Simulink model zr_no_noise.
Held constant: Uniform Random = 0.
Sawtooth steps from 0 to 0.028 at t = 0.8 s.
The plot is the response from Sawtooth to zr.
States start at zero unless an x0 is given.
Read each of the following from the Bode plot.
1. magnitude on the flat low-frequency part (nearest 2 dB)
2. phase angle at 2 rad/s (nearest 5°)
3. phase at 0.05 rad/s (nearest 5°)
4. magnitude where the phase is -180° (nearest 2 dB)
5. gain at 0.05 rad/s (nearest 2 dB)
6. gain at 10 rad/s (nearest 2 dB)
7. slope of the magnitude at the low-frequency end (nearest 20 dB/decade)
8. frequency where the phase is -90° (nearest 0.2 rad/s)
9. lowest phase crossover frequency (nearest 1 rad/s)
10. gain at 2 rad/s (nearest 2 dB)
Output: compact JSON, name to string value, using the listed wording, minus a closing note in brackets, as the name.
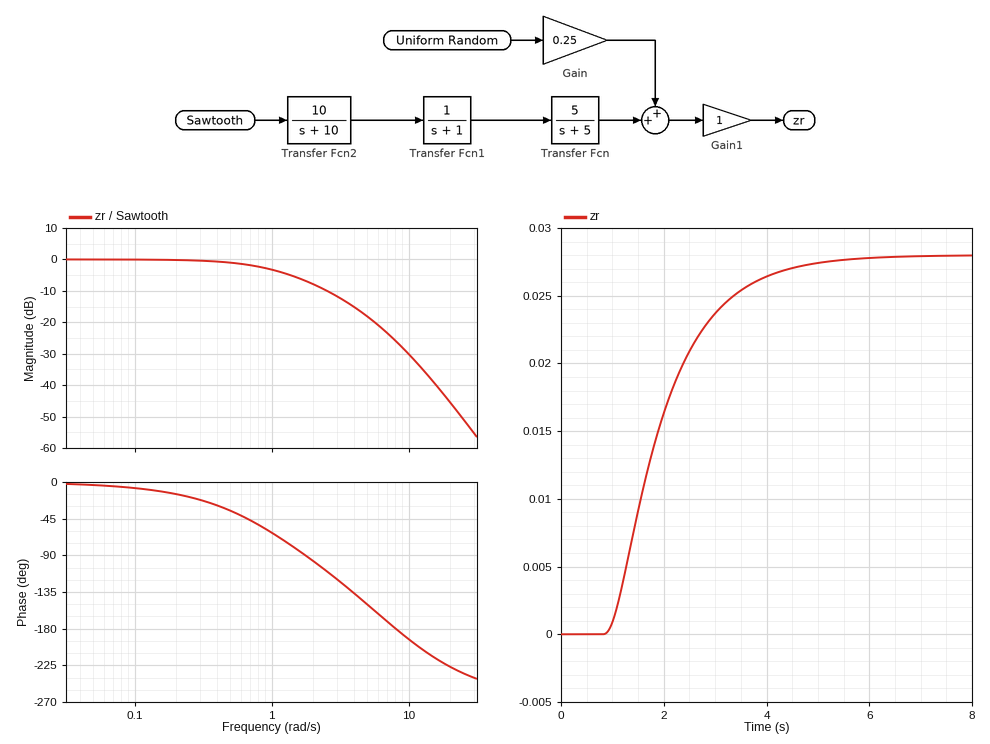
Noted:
{"magnitude on the flat low-frequency part": "0 dB", "phase angle at 2 rad/s": "-95°", "phase at 0.05 rad/s": "-5°", "magnitude where the phase is -180°": "-26 dB", "gain at 0.05 rad/s": "0 dB", "gain at 10 rad/s": "-30 dB", "slope of the magnitude at the low-frequency end": "0 dB/decade", "frequency where the phase is -90°": "1.8 rad/s", "lowest phase crossover frequency": "8 rad/s", "gain at 2 rad/s": "-8 dB"}
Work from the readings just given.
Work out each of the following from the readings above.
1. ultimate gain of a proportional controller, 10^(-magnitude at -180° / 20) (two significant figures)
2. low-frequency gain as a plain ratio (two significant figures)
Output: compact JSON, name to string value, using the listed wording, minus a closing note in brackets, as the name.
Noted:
{"ultimate gain of a proportional controller, 10^(-magnitude at -180° / 20)": "20", "low-frequency gain as a plain ratio": "1.0"}
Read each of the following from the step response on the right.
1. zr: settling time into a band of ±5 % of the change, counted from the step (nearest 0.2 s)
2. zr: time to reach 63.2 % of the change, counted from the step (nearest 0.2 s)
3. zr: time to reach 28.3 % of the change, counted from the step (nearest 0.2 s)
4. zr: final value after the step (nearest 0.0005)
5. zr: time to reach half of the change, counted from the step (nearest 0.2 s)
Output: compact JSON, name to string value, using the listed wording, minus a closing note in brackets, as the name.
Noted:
{"zr: settling time into a band of ±5 % of the change, counted from the step": "3.4 s", "zr: time to reach 63.2 % of the change, counted from the step": "1.4 s", "zr: time to reach 28.3 % of the change, counted from the step": "0.6 s", "zr: final value after the step": "0.0280", "zr: time to reach half of the change, counted from the step": "1.0 s"}
